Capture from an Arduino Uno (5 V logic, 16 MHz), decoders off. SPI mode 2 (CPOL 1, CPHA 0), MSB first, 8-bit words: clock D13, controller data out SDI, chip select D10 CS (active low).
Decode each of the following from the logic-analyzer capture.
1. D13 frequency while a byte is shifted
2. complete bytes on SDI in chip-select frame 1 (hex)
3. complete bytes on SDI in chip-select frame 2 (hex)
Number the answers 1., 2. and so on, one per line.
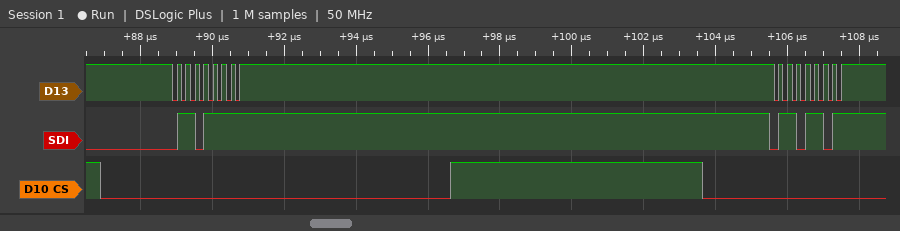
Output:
1. 4 MHz
2. 0x6F
3. 0x6D
